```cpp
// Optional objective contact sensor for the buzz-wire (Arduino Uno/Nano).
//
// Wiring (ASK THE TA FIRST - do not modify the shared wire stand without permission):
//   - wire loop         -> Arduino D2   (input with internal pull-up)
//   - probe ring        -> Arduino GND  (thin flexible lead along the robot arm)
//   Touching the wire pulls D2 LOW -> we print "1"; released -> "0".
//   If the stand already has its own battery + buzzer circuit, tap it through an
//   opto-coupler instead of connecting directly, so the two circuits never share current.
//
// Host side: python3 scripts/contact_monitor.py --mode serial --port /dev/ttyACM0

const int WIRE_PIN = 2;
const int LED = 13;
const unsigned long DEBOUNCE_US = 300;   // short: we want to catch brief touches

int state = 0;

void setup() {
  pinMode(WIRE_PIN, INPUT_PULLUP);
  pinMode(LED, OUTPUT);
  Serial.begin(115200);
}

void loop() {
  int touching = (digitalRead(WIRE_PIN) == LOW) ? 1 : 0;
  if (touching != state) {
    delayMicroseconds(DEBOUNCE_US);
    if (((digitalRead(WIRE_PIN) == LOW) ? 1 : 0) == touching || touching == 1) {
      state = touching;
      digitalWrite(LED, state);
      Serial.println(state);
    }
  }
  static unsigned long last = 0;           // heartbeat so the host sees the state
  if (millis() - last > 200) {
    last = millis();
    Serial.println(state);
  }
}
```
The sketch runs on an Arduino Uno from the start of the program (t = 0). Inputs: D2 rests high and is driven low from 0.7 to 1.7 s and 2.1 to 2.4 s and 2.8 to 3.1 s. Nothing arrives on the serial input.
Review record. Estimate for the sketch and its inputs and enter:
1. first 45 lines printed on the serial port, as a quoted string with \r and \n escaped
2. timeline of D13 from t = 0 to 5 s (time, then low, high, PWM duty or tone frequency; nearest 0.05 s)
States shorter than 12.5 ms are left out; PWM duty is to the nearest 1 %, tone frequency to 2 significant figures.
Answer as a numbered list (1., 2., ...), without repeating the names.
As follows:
1. "0\r\n0\r\n0\r\n1\r\n1\r\n1\r\n1\r\n1\r\n1\r\n0\r\n0\r\n0\r\n1\r\n1\r\n0\r\n0\r\n0\r\n1\r\n1\r\n1\r\n0\r\n0\r\n0\r\n0\r\n0\r\n0\r\n0\r\n0\r\n0\r\n0\r\n0\r\n0\r\n0\r\n0\r\n0\r\n0\r\n0\r\n0\r\n0\r\n0\r\n0\r\n0\r\n0\r\n0\r\n0\r\n"
2. 0 s low; 0.7 s high; 1.7 s low; 2.1 s high; 2.4 s low; 2.8 s high; 3.1 s low
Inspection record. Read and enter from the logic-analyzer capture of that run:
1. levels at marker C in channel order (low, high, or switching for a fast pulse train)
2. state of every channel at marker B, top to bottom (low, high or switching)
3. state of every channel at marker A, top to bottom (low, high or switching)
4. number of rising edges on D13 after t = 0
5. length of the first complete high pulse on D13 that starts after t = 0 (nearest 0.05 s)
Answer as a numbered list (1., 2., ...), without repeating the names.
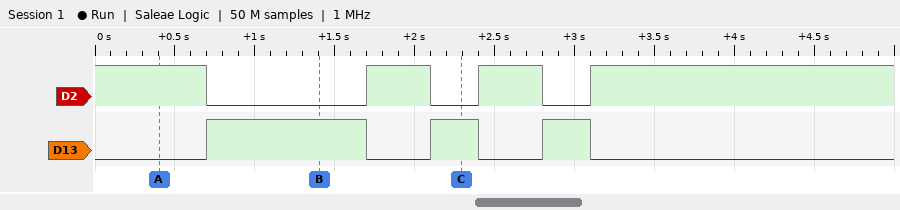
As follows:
1. D2 low, D13 high
2. D2 low, D13 high
3. D2 high, D13 low
4. 3
5. 1.00 s
